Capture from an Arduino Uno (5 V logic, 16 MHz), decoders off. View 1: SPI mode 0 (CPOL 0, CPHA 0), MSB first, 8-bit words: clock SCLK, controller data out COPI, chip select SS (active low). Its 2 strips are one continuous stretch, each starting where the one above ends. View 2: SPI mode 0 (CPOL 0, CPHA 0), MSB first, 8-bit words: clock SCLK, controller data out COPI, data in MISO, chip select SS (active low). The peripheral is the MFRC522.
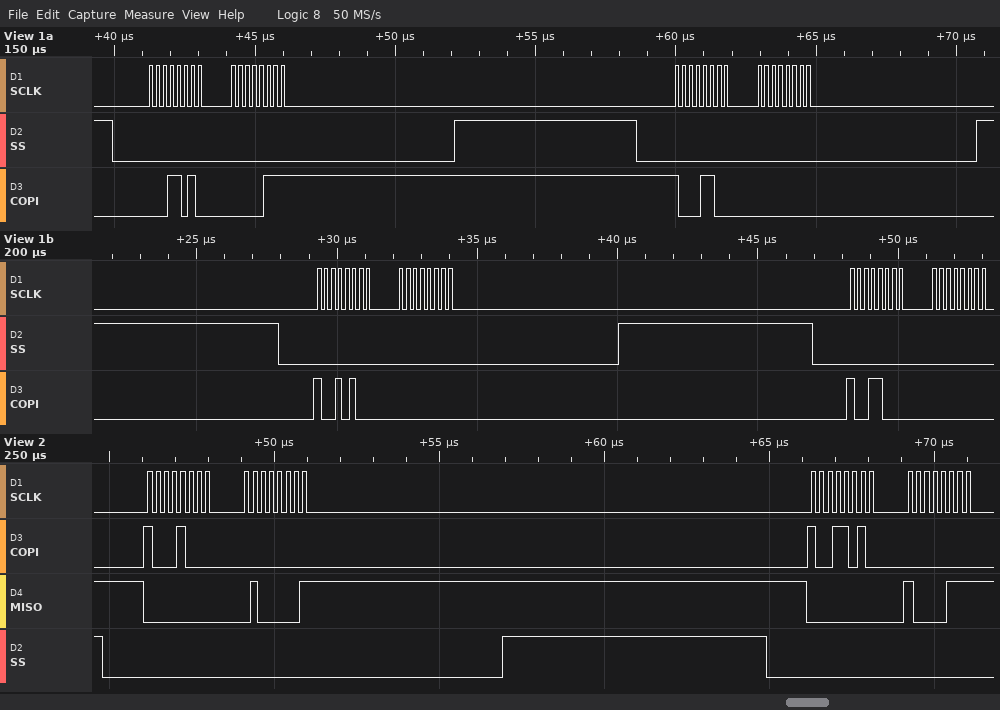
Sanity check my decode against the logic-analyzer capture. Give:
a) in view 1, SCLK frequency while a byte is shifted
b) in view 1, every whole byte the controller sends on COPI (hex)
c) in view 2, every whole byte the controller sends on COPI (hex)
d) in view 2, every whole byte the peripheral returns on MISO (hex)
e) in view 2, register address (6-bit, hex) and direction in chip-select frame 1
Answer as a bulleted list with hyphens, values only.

- 4 MHz
- 1A 07 8C 00 94 00 98 00
- 88 00 9A 00
- 00 41 00 87
- 0x04 read
